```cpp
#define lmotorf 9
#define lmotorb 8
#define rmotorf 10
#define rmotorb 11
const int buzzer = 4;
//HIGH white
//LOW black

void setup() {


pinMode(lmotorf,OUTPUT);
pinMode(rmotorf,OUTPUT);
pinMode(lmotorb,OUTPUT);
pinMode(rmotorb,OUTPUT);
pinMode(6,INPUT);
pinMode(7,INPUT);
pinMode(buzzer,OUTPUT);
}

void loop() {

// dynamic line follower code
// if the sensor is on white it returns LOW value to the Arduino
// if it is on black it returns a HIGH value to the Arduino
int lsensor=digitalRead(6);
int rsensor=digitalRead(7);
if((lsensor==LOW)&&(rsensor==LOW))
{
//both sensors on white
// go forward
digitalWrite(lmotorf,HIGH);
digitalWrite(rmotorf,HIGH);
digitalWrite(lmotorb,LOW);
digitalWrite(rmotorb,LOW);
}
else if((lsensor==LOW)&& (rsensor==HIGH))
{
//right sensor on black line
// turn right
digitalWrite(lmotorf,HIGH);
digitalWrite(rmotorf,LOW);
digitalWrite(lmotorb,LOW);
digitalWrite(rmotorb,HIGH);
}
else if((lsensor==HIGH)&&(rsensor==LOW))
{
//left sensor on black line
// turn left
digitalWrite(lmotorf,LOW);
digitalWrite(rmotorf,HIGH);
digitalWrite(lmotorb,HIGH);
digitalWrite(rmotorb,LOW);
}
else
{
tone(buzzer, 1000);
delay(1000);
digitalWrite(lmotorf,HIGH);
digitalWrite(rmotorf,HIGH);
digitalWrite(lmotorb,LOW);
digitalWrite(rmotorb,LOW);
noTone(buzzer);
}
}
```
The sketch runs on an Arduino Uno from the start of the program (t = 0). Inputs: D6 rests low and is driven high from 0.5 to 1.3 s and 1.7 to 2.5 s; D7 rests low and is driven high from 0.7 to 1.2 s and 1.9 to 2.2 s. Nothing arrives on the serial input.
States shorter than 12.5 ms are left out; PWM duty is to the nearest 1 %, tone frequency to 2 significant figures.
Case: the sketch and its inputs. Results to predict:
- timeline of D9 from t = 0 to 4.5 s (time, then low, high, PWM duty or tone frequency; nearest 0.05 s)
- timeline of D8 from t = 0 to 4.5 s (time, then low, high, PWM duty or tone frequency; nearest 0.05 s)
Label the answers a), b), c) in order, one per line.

a) 0 s high; 0.5 s low; 2.9 s high
b) 0 s low; 0.5 s high; 2.9 s low
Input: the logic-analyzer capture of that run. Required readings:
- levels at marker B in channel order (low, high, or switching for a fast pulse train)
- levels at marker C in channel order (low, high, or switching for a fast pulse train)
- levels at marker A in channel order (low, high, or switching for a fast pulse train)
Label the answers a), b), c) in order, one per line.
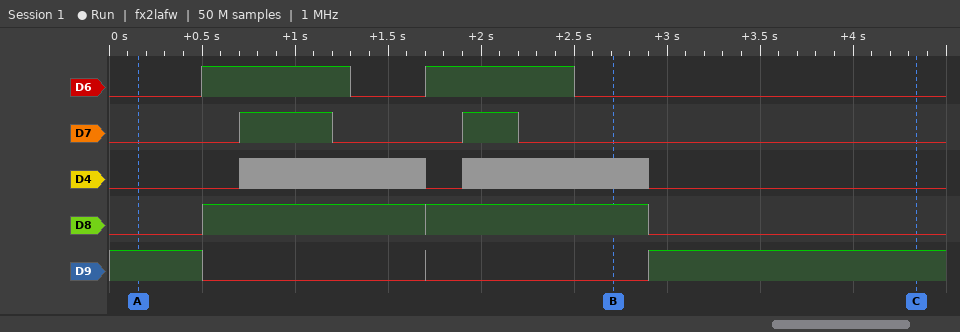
a) D6 low, D7 low, D4 switching, D8 high, D9 low
b) D6 low, D7 low, D4 low, D8 low, D9 high
c) D6 low, D7 low, D4 low, D8 low, D9 high
